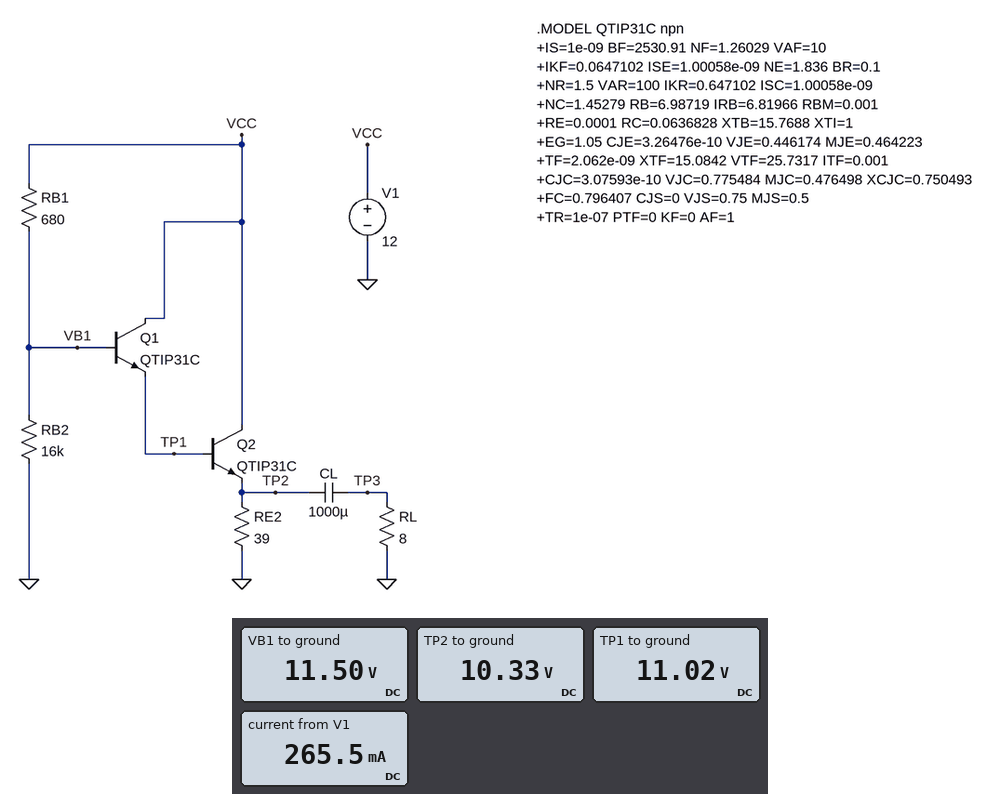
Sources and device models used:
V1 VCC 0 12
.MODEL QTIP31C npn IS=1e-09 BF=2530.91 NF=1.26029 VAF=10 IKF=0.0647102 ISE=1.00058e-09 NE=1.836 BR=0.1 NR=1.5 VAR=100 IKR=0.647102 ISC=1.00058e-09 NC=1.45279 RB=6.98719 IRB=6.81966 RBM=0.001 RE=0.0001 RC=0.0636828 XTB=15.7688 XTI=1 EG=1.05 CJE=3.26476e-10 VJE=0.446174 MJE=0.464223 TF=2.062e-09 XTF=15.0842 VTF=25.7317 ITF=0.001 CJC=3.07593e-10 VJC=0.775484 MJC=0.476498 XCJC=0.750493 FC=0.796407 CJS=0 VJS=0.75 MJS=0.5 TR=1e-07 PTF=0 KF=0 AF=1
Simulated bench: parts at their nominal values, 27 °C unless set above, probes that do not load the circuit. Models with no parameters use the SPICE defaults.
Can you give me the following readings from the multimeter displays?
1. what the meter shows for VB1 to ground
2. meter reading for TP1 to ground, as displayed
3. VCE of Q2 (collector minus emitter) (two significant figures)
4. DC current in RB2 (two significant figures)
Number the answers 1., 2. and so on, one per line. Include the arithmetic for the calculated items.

1. 11.50 V
2. 11.02 V
3. 12 V - 10.33 V = 1.7 V
4. (11.5 V) / 16 kΩ = 720 µA
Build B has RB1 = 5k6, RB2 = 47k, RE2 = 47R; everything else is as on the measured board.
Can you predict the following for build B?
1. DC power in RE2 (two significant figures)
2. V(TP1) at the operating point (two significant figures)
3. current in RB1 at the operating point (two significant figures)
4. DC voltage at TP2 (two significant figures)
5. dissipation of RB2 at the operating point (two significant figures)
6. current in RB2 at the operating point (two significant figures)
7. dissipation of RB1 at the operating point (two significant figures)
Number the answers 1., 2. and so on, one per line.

1. 1.9 W
2. 10 V
3. 240 µA
4. 9.5 V
5. 2.4 mW
6. 230 µA
7. 330 µW
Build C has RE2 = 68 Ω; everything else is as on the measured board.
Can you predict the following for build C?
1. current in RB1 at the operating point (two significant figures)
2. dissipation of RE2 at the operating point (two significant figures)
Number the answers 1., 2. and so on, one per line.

1. 730 µA
2. 1.6 W
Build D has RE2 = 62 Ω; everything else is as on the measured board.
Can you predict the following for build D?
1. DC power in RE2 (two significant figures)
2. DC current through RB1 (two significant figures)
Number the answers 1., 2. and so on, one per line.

1. 1.7 W
2. 730 µA
